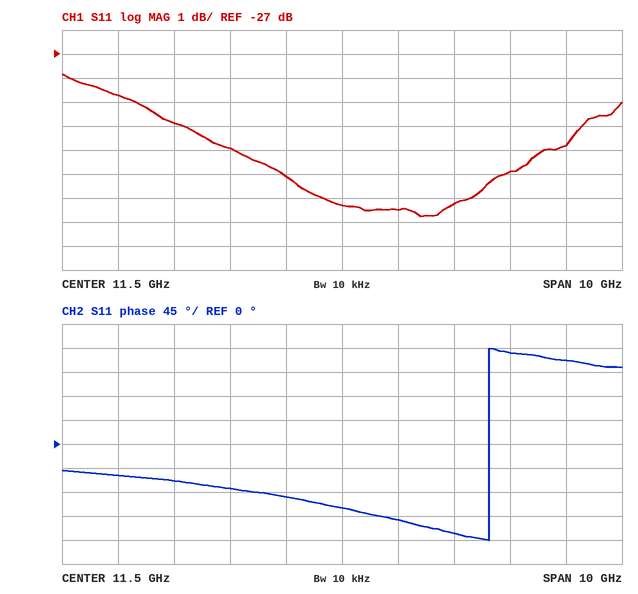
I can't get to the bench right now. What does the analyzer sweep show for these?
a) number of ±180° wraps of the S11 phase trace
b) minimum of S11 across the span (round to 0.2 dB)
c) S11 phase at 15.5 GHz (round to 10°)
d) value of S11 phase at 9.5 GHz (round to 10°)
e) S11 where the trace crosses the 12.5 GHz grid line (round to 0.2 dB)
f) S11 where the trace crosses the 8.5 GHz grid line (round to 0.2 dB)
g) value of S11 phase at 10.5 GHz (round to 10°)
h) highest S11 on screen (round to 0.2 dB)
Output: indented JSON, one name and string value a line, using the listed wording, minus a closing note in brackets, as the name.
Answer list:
{
  "number of ±180° wraps of the S11 phase trace": "1",
  "minimum of S11 across the span": "-33.8 dB",
  "S11 phase at 15.5 GHz": "160°",
  "value of S11 phase at 9.5 GHz": "-80°",
  "S11 where the trace crosses the 12.5 GHz grid line": "-33.4 dB",
  "S11 where the trace crosses the 8.5 GHz grid line": "-29.8 dB",
  "value of S11 phase at 10.5 GHz": "-100°",
  "highest S11 on screen": "-27.8 dB"
}
